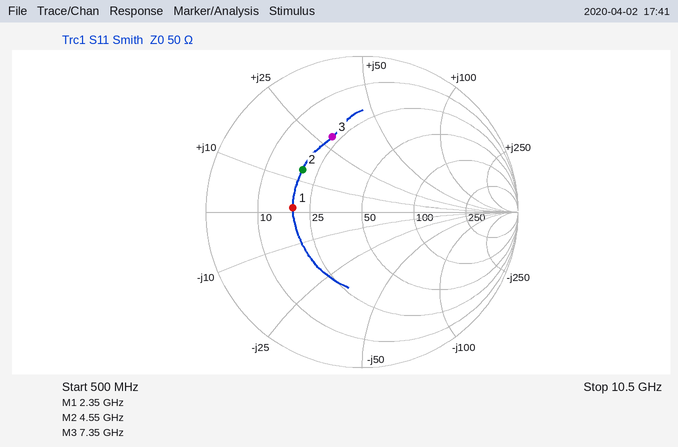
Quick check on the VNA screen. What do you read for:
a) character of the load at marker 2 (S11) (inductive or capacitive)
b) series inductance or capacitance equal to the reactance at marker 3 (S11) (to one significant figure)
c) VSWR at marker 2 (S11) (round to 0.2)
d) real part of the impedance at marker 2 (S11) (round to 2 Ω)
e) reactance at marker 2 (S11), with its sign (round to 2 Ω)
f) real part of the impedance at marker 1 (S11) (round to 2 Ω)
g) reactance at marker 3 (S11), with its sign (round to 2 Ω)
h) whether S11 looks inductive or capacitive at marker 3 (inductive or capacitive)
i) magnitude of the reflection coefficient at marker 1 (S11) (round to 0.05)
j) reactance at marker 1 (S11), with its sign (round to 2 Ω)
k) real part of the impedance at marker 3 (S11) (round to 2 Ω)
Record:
inductive
600 pH
2.8
20 Ω
+14 Ω
20 Ω
+30 Ω
inductive
0.45
+2 Ω
22 Ω
